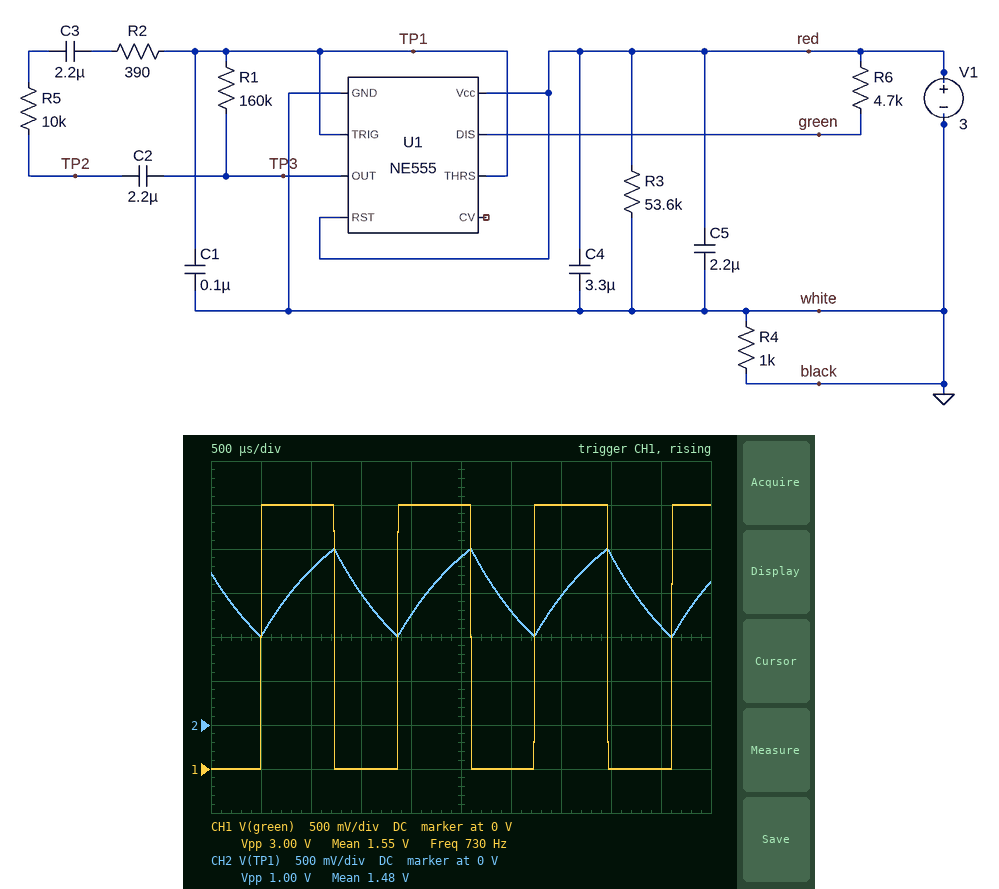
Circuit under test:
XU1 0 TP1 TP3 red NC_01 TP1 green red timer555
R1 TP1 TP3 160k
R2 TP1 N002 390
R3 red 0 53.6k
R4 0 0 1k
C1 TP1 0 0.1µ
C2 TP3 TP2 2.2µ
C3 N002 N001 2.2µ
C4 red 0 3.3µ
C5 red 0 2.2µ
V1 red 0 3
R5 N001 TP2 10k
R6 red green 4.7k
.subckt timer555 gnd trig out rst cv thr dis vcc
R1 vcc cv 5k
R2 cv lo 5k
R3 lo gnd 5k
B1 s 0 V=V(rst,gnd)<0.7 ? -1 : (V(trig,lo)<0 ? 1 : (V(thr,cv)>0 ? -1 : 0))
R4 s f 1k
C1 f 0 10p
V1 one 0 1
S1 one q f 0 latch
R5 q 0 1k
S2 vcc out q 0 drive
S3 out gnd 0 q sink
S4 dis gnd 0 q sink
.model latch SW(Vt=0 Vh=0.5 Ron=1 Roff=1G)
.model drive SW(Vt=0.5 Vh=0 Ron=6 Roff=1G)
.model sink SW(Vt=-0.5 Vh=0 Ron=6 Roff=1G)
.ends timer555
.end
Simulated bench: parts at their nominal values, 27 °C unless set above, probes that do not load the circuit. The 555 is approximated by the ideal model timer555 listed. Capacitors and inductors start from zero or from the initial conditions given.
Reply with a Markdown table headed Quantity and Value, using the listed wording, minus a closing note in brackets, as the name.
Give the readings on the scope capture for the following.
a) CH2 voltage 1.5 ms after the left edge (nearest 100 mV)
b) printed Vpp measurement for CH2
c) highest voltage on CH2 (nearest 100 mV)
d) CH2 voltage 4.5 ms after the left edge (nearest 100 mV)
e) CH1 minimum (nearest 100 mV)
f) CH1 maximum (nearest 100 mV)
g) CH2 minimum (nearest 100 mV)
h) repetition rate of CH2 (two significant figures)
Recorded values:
| Quantity | Value |
|---|---|
| CH2 voltage 1.5 ms after the left edge | 1.5 V |
| printed Vpp measurement for CH2 | 1.00 V |
| highest voltage on CH2 | 2.0 V |
| CH2 voltage 4.5 ms after the left edge | 1.1 V |
| CH1 minimum | 0 V |
| CH1 maximum | 3.0 V |
| CH2 minimum | 1.0 V |
| repetition rate of CH2 | 730 Hz |
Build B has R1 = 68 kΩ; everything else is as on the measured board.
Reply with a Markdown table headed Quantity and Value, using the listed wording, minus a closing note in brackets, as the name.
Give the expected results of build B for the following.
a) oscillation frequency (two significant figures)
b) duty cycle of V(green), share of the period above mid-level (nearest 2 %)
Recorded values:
| Quantity | Value |
|---|---|
| oscillation frequency | 790 Hz |
| duty cycle of V(green), share of the period above mid-level | 52 % |
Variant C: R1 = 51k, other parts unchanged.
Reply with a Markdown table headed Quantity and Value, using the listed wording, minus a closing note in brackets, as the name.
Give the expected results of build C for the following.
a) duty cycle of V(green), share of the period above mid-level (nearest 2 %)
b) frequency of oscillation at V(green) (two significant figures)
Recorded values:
| Quantity | Value |
|---|---|
| duty cycle of V(green), share of the period above mid-level | 52 % |
| frequency of oscillation at V(green) | 830 Hz |
